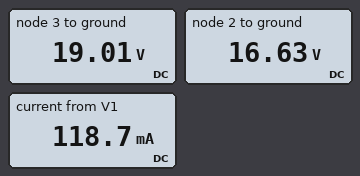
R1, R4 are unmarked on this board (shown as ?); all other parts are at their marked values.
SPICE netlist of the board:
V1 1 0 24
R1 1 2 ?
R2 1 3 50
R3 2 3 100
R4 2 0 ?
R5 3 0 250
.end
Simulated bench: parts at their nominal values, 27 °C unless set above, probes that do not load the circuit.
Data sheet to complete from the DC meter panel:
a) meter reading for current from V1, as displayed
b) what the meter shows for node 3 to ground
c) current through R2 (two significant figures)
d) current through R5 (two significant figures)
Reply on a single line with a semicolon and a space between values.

118.7 mA; 19.01 V; 100 mA; 76 mA
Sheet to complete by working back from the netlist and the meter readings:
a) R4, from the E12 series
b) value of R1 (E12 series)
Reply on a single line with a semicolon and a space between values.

390 Ω; 390 Ω
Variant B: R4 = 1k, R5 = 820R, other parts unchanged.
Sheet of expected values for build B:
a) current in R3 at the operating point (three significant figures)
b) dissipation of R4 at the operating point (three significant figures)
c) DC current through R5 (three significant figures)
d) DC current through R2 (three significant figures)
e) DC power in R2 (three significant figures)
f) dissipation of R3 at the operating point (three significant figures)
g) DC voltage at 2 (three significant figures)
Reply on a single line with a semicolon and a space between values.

12.5 mA; 432 mW; 26.9 mA; 39.4 mA; 77.6 mW; 15.7 mW; 20.8 V
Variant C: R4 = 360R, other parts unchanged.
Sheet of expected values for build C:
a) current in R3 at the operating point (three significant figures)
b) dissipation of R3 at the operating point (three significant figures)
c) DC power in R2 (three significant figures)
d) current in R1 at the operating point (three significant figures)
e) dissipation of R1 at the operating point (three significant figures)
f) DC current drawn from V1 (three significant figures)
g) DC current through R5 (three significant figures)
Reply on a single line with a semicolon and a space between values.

25.8 mA; 66.5 mW; 515 mW; 19.6 mA; 150 mW; 121 mA; 75.7 mA
